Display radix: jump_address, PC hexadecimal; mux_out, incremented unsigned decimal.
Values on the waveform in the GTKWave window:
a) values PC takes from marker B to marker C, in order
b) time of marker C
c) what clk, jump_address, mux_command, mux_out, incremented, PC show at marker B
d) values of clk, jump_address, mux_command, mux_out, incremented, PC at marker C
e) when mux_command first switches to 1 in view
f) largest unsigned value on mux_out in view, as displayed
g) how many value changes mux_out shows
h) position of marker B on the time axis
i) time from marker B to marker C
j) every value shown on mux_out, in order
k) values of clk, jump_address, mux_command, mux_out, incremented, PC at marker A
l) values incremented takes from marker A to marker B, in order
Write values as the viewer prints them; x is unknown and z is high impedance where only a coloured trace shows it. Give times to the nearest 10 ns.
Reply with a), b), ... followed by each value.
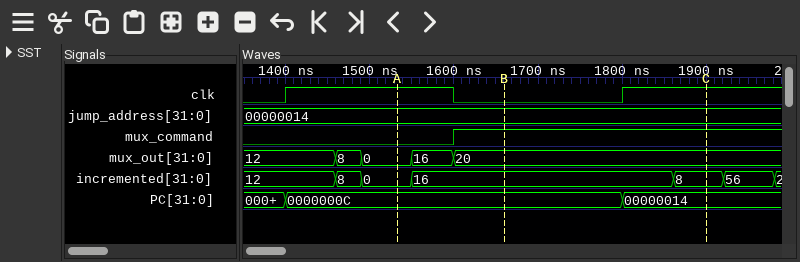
a) 0000000C, 00000014
b) 1900 ns
c) clk=0, jump_address=00000014, mux_command=1, mux_out=20, incremented=16, PC=0000000C
d) clk=1, jump_address=00000014, mux_command=1, mux_out=20, incremented=8, PC=00000014
e) 1600 ns
f) 20
g) 4
h) 1660 ns
i) 240 ns
j) 12, 8, 0, 16, 20
k) clk=1, jump_address=00000014, mux_command=0, mux_out=0, incremented=0, PC=0000000C
l) 0, 16
